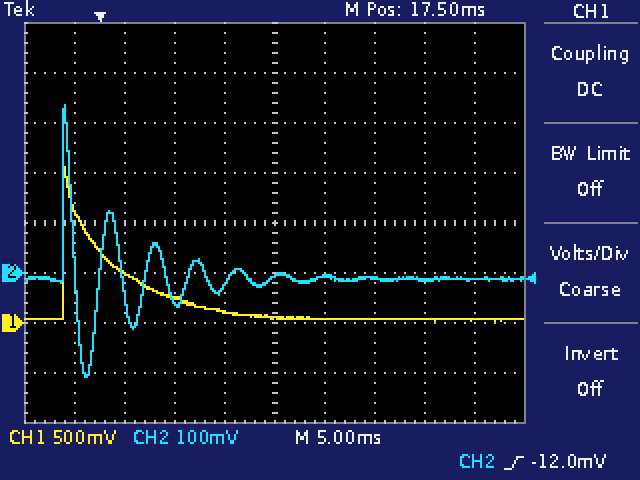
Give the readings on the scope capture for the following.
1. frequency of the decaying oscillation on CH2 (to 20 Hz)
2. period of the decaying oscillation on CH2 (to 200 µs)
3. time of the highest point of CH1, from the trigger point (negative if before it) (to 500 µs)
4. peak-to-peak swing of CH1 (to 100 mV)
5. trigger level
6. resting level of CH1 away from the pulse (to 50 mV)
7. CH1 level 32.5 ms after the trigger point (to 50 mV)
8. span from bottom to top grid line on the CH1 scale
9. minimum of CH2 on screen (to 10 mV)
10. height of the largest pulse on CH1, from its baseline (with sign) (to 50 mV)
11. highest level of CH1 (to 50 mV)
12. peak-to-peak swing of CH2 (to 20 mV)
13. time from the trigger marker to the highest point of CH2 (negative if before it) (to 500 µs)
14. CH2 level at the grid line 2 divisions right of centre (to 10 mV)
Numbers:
240 Hz
4.2 ms
-3.5 ms
1.50 V
-12.0 mV
50 mV
50 mV
4 V
-210 mV
+1.50 V
1.55 V
540 mV
-3.5 ms
-10 mV
